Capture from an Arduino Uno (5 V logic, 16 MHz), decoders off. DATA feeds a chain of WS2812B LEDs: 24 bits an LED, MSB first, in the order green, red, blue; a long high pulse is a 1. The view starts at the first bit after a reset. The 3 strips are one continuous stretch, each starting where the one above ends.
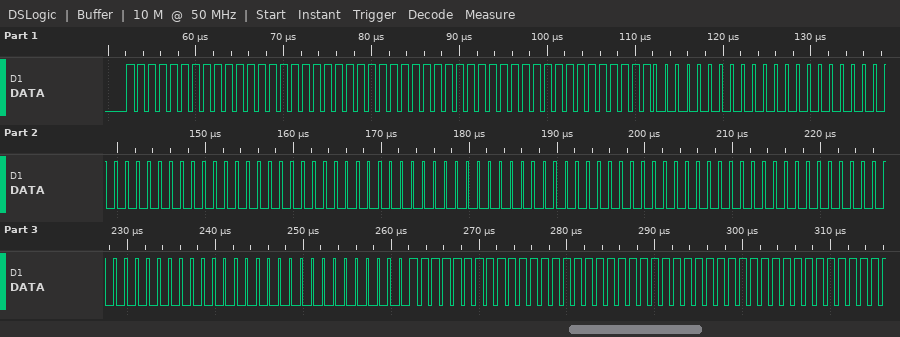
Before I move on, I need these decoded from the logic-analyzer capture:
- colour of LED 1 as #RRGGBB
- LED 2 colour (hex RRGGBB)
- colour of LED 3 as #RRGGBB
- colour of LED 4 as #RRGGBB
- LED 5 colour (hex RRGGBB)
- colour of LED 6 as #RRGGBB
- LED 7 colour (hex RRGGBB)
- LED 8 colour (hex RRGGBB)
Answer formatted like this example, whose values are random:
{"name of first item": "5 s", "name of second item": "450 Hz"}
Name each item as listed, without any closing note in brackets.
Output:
{"colour of LED 1 as #RRGGBB": "#FFFFFF", "LED 2 colour": "#FFFFFF", "colour of LED 3 as #RRGGBB": "#000000", "colour of LED 4 as #RRGGBB": "#000000", "LED 5 colour": "#000000", "colour of LED 6 as #RRGGBB": "#000000", "LED 7 colour": "#000000", "LED 8 colour": "#FFFFFF"}
